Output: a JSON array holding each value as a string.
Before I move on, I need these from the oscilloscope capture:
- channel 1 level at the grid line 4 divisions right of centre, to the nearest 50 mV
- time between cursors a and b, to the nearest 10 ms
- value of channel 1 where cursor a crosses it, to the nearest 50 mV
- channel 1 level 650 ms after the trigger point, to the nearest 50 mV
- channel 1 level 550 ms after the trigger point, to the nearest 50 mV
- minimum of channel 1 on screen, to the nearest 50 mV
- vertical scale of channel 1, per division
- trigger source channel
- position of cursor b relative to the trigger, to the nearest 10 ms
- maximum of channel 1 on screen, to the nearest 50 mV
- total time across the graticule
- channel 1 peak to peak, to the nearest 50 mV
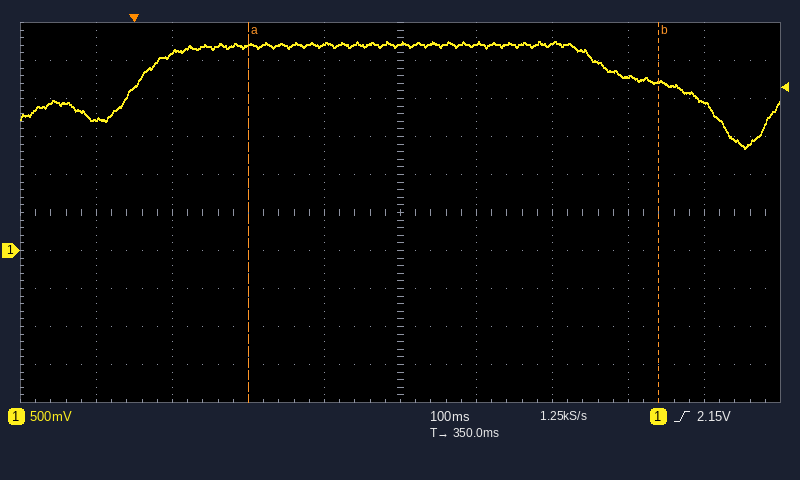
["1.95 V", "540 ms", "2.70 V", "2.30 V", "2.70 V", "1.35 V", "500 mV", "channel 1", "+690 ms", "2.75 V", "1 s", "1.40 V"]
